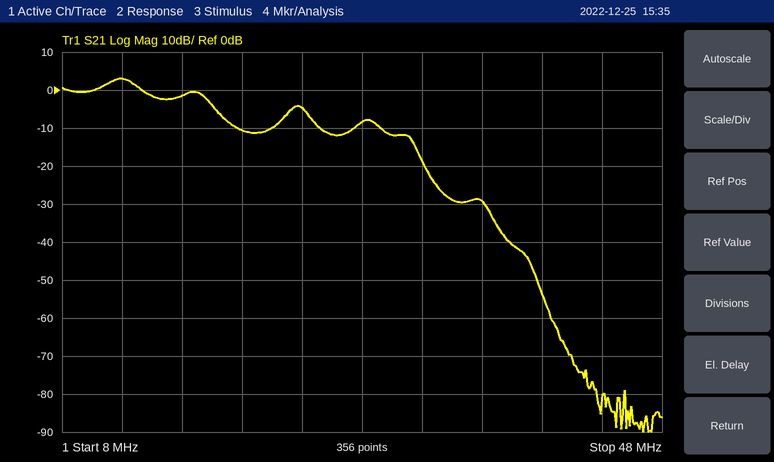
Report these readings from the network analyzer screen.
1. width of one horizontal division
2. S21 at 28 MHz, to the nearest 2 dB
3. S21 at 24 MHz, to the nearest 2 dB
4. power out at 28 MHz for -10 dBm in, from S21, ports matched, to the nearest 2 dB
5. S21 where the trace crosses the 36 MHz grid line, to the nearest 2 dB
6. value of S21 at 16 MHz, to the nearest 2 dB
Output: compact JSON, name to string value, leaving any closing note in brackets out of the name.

{"width of one horizontal division": "4 MHz", "S21 at 28 MHz, to the nearest 2 dB": "-8 dB", "S21 at 24 MHz, to the nearest 2 dB": "-4 dB", "power out at 28 MHz for -10 dBm in, from S21, ports matched, to the nearest 2 dB": "-18 dBm", "S21 where the trace crosses the 36 MHz grid line, to the nearest 2 dB": "-30 dB", "value of S21 at 16 MHz, to the nearest 2 dB": "-2 dB"}
